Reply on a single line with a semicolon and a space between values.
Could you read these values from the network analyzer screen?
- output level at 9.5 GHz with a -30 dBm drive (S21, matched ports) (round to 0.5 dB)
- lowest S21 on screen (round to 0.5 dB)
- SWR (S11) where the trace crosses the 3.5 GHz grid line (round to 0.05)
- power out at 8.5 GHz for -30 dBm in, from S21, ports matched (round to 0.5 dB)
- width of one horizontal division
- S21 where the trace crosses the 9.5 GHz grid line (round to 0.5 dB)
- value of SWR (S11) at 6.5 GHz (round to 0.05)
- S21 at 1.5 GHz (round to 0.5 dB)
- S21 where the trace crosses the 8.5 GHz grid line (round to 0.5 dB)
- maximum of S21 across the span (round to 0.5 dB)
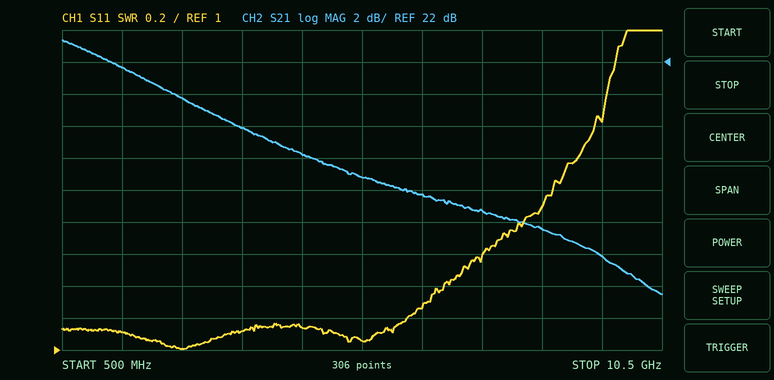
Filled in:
-20.0 dBm; 7.5 dB; 1.10; -18.5 dBm; 1 GHz; 10.0 dB; 1.25; 21.5 dB; 11.5 dB; 23.5 dB
